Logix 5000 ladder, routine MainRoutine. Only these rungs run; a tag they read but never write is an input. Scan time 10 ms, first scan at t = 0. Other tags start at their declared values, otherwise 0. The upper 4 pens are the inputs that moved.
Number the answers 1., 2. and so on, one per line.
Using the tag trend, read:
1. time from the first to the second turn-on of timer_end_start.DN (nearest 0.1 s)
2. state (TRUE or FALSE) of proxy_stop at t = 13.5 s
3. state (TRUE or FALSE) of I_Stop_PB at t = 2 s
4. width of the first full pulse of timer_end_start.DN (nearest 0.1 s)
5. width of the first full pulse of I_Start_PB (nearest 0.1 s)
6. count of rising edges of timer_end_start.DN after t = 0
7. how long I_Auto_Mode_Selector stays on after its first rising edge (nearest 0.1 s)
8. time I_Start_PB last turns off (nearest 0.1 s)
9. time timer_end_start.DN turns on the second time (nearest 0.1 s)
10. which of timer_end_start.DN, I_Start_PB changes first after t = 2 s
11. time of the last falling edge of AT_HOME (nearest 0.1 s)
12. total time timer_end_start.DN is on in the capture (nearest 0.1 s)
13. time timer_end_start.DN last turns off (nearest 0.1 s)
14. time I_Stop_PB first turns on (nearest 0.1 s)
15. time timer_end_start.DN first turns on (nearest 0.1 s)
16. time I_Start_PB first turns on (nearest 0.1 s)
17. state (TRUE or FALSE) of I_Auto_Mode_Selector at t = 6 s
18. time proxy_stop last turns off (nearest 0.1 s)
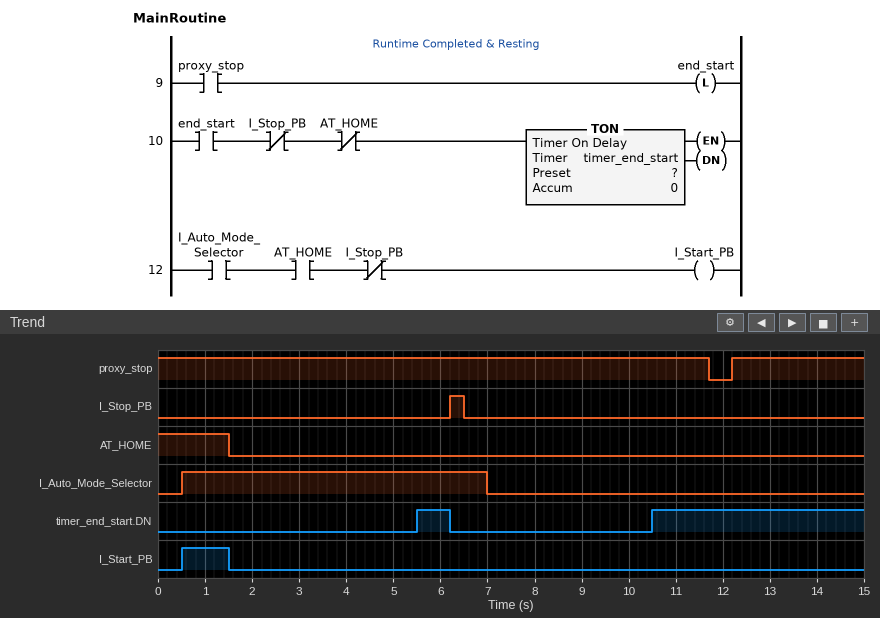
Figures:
1. 5.0 s
2. TRUE
3. FALSE
4. 0.7 s
5. 1.0 s
6. 2
7. 6.5 s
8. 1.5 s
9. 10.5 s
10. timer_end_start.DN
11. 1.5 s
12. 5.2 s
13. 6.2 s
14. 6.2 s
15. 5.5 s
16. 0.5 s
17. TRUE
18. 11.7 s
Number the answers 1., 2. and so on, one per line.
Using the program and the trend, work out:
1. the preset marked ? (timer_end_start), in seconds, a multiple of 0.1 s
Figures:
1. 4.0 s
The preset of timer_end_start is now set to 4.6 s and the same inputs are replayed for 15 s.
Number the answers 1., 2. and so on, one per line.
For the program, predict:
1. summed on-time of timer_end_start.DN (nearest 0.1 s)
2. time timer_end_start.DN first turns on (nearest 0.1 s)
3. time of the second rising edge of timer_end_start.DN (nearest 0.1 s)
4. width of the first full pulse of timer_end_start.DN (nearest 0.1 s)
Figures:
1. 4.0 s
2. 6.1 s
3. 11.1 s
4. 0.1 s
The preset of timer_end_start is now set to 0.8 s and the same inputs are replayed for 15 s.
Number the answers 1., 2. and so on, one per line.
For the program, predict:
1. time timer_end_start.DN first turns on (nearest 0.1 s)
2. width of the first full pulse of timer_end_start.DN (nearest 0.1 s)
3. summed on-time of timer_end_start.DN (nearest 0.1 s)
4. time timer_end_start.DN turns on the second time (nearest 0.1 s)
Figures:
1. 2.3 s
2. 3.9 s
3. 11.6 s
4. 7.3 s
